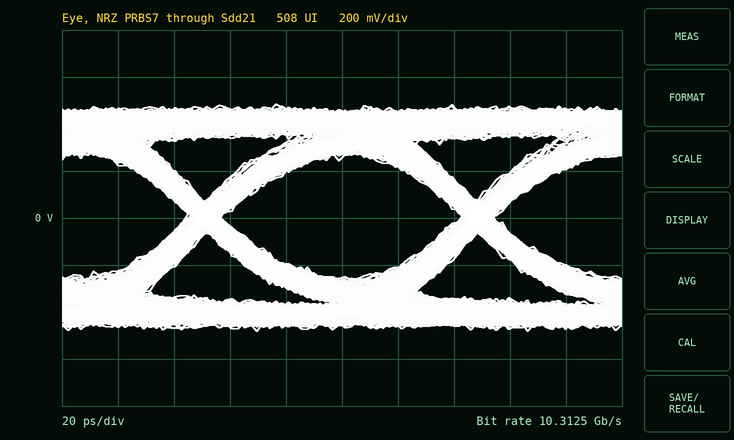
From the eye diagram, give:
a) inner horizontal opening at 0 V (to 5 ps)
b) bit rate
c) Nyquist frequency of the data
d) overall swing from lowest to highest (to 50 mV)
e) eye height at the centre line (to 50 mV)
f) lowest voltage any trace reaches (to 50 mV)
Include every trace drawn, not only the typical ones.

85 ps
10.3125 Gb/s
5.15625 GHz
950 mV
500 mV
-500 mV
